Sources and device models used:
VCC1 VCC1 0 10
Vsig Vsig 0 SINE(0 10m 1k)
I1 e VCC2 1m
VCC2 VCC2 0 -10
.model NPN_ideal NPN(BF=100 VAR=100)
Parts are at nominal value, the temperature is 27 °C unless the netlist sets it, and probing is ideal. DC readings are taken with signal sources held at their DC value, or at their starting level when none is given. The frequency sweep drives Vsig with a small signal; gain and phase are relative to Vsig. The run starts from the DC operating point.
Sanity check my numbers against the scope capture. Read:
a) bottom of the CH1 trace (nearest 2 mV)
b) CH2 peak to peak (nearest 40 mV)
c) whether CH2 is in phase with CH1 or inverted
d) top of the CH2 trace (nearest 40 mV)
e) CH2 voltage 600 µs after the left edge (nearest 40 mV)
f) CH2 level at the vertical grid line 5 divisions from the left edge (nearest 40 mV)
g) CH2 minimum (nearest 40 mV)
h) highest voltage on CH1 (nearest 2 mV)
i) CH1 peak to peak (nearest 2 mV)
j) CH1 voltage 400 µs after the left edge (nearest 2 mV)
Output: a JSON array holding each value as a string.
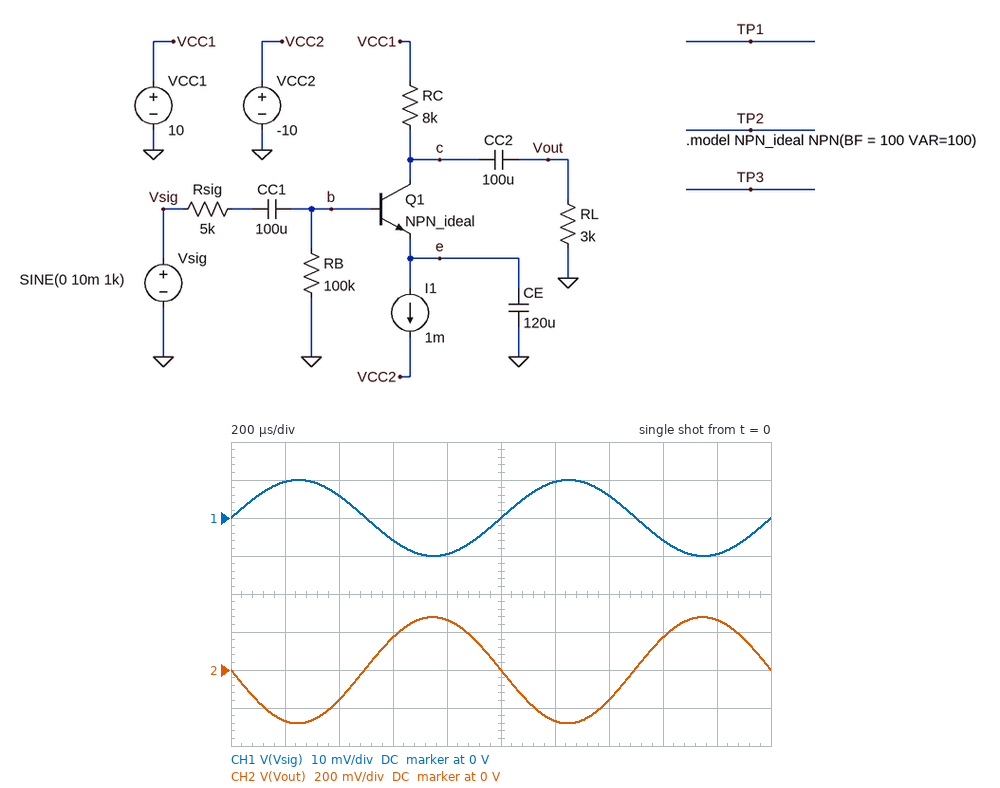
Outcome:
["-10 mV", "560 mV", "inverted", "280 mV", "160 mV", "0 V", "-280 mV", "10 mV", "20 mV", "6 mV"]
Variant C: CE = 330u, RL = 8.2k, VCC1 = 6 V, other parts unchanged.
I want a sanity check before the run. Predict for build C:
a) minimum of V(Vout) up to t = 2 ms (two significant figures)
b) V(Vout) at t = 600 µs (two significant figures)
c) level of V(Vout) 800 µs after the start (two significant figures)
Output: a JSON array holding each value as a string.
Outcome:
["-13 mV", "13 mV", "26 mV"]
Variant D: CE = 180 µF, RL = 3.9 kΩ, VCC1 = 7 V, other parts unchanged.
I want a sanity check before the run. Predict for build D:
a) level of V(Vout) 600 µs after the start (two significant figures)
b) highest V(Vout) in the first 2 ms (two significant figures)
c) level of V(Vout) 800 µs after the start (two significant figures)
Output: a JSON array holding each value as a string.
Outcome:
["200 mV", "330 mV", "320 mV"]
